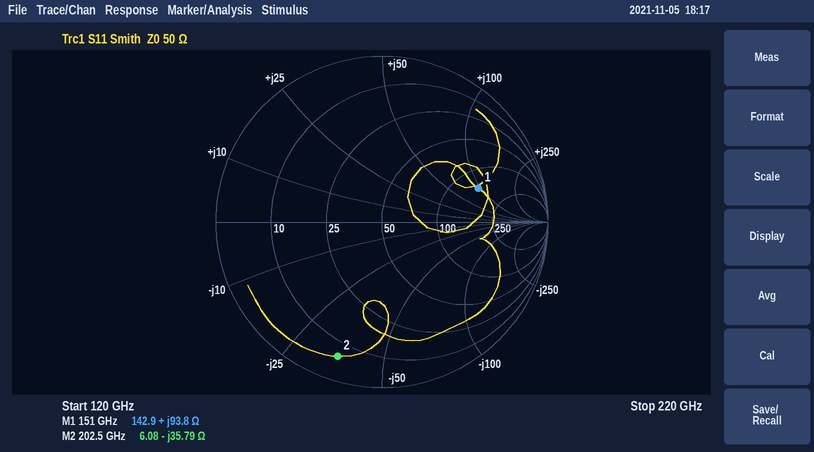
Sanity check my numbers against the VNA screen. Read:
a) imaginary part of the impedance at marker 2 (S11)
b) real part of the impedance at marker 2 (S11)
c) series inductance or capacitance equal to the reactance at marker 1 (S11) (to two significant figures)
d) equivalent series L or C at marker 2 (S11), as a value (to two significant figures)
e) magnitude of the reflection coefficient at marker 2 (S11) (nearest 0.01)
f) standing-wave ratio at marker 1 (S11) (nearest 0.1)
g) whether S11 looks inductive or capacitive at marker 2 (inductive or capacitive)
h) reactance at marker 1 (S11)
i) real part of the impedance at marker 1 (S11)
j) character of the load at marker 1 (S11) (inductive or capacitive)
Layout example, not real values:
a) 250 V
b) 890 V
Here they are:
a) -35.79 Ω
b) 6.08 Ω
c) 99 pH
d) 22 fF
e) 0.85
f) 4.2
g) capacitive
h) +93.8 Ω
i) 142.9 Ω
j) inductive
